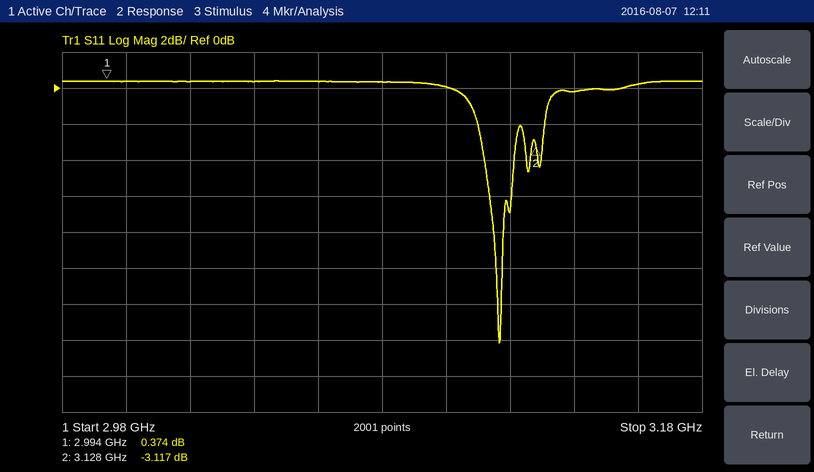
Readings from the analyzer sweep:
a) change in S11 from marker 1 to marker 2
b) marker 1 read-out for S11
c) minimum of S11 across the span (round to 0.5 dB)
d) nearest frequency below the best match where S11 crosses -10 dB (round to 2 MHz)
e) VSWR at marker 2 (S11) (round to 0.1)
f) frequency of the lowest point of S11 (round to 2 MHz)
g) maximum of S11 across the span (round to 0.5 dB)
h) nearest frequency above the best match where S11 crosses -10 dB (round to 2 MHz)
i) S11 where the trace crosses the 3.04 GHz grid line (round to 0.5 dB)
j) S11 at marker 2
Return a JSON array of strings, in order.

["-3.491 dB", "0.374 dB", "-14.0 dB", "3.116 GHz", "5.6", "3.116 GHz", "0.5 dB", "3.118 GHz", "0.5 dB", "-3.117 dB"]
